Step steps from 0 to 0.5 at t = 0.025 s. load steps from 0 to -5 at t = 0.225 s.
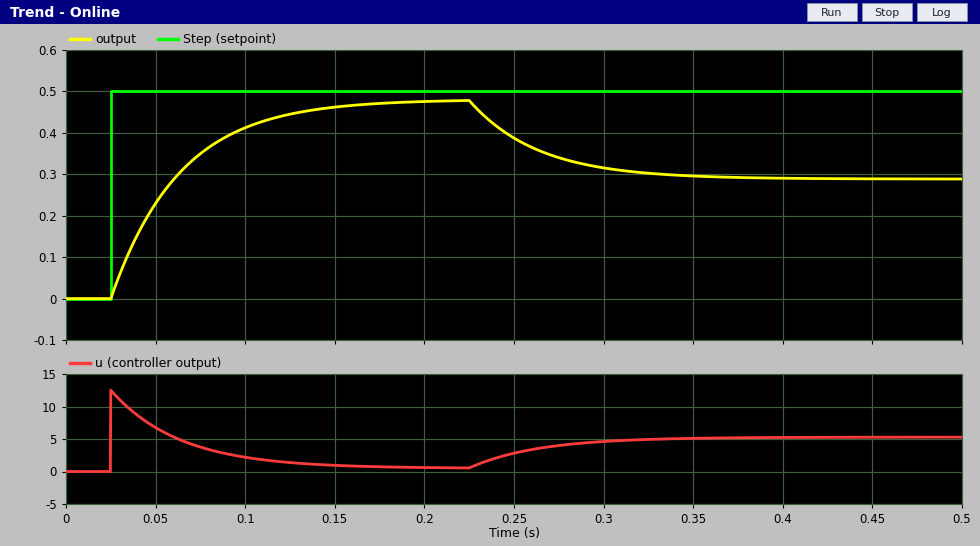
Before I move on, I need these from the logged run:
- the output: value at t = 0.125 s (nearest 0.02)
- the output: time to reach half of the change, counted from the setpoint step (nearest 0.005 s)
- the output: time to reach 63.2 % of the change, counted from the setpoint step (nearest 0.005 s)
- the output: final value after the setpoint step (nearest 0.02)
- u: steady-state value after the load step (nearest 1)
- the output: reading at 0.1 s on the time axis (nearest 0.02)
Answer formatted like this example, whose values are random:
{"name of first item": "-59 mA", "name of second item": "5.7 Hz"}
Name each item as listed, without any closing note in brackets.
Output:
{"the output: value at t = 0.125 s": "0.44", "the output: time to reach half of the change, counted from the setpoint step": "0.025 s", "the output: time to reach 63.2 % of the change, counted from the setpoint step": "0.040 s", "the output: final value after the setpoint step": "0.48", "u: steady-state value after the load step": "5", "the output: reading at 0.1 s on the time axis": "0.42"}
